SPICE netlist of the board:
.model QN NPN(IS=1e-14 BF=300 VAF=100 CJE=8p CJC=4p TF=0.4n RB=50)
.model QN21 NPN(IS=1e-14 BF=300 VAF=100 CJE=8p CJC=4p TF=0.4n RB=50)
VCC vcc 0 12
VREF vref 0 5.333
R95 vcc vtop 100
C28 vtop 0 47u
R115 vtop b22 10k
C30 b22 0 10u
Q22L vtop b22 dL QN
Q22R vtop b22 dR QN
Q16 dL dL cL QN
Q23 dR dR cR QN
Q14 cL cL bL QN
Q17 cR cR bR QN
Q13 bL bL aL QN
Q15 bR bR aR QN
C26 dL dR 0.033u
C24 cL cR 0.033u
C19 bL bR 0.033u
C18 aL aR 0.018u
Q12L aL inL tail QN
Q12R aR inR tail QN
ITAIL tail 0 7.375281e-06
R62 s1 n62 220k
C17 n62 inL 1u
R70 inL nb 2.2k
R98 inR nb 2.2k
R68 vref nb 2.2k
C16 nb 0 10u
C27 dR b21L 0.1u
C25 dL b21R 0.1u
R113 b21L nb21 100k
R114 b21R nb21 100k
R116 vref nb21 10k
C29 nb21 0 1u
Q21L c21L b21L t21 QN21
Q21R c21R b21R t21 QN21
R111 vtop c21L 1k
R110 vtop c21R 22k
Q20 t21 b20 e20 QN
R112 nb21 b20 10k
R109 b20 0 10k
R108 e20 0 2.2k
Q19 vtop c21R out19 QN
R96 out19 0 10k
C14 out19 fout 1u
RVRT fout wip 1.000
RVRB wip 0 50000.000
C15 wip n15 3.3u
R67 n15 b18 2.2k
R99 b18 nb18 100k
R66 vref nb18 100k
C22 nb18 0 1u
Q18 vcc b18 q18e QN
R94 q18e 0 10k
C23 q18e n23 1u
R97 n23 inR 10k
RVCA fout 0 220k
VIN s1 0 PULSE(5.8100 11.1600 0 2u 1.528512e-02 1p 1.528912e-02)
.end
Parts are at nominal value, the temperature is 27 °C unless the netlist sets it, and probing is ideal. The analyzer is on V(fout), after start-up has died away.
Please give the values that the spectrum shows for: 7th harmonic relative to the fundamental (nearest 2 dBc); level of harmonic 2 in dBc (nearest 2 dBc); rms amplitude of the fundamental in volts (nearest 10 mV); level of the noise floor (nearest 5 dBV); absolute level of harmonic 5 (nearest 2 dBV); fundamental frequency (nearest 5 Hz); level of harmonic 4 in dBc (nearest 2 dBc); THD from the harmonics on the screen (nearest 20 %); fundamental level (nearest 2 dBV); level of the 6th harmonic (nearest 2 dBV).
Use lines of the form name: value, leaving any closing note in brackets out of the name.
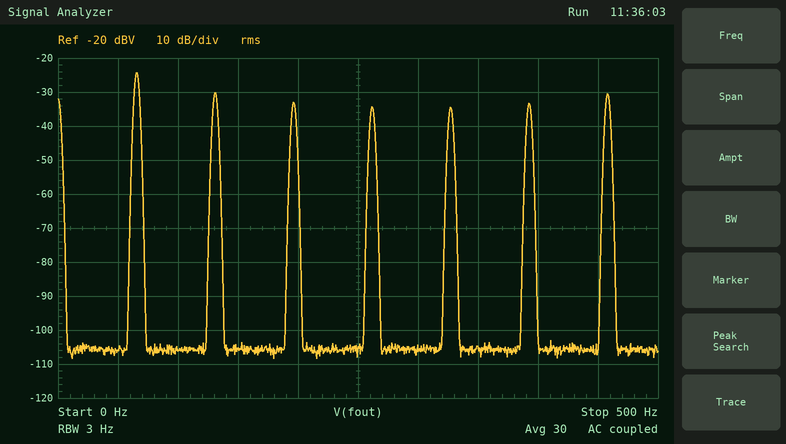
7th harmonic relative to the fundamental: -6 dBc
level of harmonic 2 in dBc: -6 dBc
rms amplitude of the fundamental in volts: 60 mV
level of the noise floor: -105 dBV
absolute level of harmonic 5: -34 dBV
fundamental frequency: 65 Hz
level of harmonic 4 in dBc: -10 dBc
THD from the harmonics on the screen: 100 %
fundamental level: -24 dBV
level of the 6th harmonic: -34 dBV
